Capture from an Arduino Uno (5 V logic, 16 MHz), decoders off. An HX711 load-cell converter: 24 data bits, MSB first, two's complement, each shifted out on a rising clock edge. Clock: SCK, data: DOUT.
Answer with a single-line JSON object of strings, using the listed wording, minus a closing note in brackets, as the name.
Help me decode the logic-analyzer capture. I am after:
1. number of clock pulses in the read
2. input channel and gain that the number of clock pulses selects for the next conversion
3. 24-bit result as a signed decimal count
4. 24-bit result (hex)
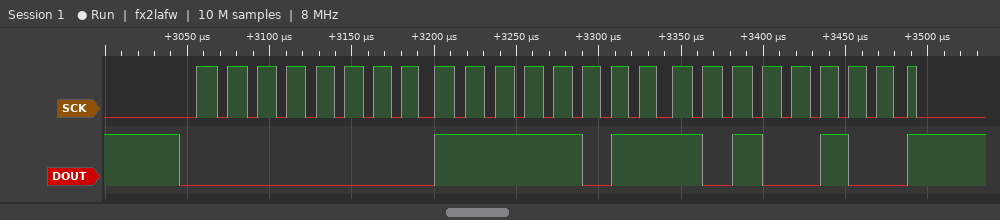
{"number of clock pulses in the read": "25", "input channel and gain that the number of clock pulses selects for the next conversion": "channel A, gain 128", "24-bit result as a signed decimal count": "64420", "24-bit result": "0x00FBA4"}
